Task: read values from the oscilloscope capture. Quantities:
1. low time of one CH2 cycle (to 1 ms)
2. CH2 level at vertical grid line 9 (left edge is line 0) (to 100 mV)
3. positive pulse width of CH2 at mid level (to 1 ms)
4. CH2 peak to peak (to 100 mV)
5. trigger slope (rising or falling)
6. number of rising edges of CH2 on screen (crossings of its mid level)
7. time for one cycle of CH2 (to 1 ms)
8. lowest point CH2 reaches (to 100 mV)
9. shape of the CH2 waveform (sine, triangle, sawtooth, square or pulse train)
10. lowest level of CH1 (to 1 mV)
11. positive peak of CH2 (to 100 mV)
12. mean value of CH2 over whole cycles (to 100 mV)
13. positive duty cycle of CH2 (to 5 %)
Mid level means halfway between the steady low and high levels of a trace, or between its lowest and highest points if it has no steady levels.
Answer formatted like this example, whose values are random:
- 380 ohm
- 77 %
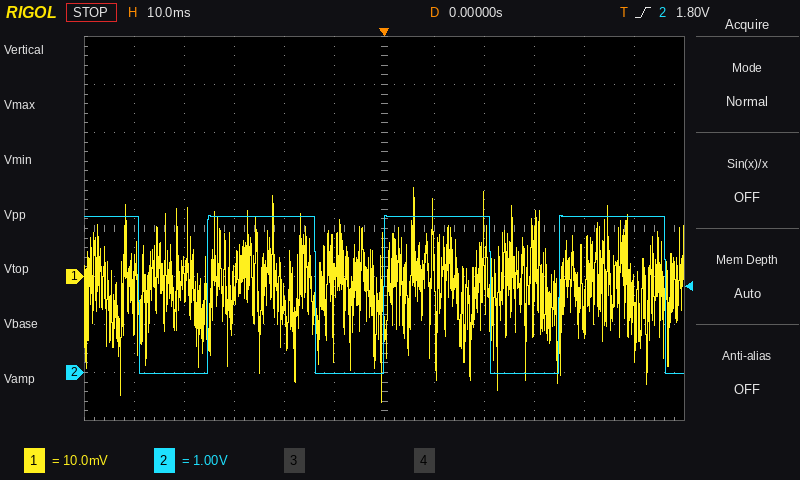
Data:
- 14 ms
- 0.0 V
- 21 ms
- 3.3 V
- rising
- 3
- 35 ms
- 0.0 V
- pulse train
- -26 mV
- 3.3 V
- 2.0 V
- 60 %
